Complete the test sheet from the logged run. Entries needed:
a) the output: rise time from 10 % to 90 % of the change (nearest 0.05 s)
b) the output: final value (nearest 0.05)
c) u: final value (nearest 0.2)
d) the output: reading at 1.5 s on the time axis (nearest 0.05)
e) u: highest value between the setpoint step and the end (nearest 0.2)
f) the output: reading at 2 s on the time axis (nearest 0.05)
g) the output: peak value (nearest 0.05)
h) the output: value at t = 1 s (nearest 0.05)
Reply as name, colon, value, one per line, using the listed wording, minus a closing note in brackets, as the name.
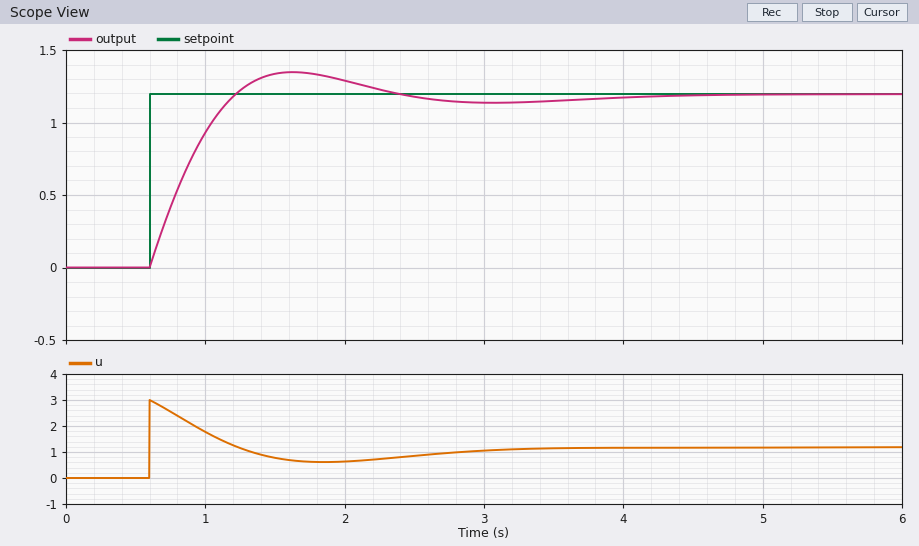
the output: rise time from 10 % to 90 % of the change: 0.45 s
the output: final value: 1.20
u: final value: 1.2
the output: reading at 1.5 s on the time axis: 1.35
u: highest value between the setpoint step and the end: 3.0
the output: reading at 2 s on the time axis: 1.30
the output: peak value: 1.35
the output: value at t = 1 s: 0.95
